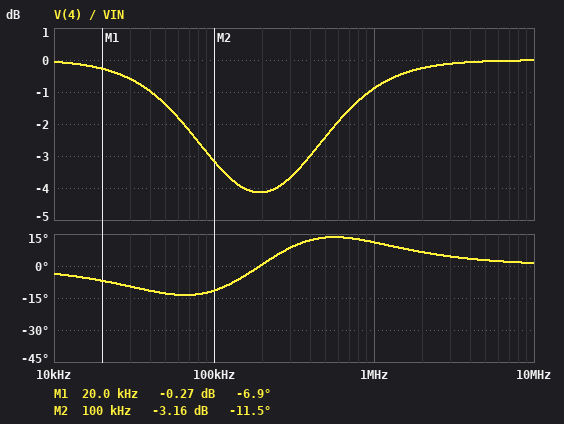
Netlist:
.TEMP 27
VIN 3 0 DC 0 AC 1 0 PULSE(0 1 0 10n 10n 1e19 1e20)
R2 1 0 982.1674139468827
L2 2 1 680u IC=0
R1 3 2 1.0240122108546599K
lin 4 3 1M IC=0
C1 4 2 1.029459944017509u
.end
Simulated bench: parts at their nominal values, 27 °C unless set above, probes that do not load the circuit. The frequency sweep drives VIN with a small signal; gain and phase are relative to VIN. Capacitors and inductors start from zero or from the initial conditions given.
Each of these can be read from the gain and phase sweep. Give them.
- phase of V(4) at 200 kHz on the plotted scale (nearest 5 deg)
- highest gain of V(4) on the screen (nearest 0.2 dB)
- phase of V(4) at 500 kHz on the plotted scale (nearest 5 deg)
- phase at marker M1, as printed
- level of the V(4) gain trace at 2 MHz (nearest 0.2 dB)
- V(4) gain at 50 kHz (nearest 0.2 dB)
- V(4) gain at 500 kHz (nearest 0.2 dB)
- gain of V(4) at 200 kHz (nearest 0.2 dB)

0 deg
0 dB
15 deg
-6.9 deg
-0.2 dB
-1.4 dB
-2.4 dB
-4.2 dB
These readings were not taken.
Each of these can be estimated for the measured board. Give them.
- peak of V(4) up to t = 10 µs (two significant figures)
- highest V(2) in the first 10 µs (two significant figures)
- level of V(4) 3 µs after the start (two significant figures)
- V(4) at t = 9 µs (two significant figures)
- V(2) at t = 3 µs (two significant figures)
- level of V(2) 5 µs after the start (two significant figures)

990 mV
990 mV
860 mV
990 mV
860 mV
940 mV
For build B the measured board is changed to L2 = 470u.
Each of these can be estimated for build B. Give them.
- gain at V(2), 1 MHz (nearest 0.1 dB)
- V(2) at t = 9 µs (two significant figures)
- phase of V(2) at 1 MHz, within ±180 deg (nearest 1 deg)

-1.5 dB
990 mV
14 deg
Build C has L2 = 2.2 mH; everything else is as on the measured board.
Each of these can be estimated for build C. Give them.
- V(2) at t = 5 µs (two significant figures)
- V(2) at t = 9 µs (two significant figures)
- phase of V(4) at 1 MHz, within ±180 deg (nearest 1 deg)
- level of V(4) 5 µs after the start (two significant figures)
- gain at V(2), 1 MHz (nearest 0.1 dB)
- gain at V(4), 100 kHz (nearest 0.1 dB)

910 mV
970 mV
4 deg
920 mV
-0.2 dB
-2.4 dB
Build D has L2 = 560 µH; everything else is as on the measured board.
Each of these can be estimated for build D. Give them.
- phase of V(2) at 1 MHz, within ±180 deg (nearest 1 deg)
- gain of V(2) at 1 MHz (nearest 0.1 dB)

13 deg
-1.2 dB
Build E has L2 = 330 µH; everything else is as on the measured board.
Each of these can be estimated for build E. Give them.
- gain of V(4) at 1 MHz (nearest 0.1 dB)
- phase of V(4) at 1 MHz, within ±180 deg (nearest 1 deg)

-2.3 dB
16 deg
